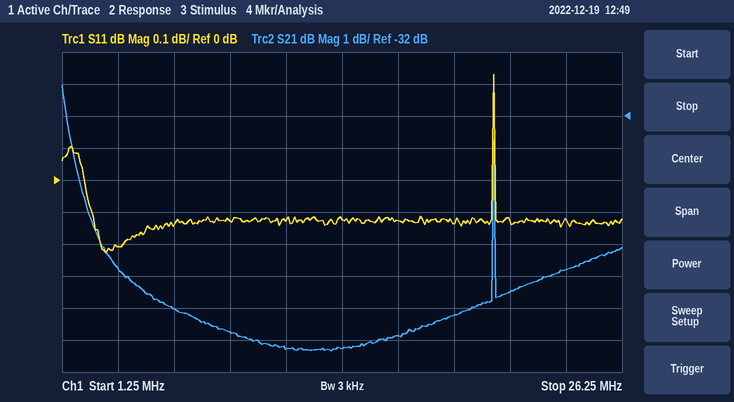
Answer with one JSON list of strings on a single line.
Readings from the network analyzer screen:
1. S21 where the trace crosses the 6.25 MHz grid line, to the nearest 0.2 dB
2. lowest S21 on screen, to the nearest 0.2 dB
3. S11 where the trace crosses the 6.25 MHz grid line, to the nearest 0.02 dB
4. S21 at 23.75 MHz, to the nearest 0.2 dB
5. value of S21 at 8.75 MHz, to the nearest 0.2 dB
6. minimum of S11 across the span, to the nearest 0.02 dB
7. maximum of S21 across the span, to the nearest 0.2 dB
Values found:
["-38.0 dB", "-39.4 dB", "-0.14 dB", "-36.8 dB", "-38.8 dB", "-0.22 dB", "-31.0 dB"]
